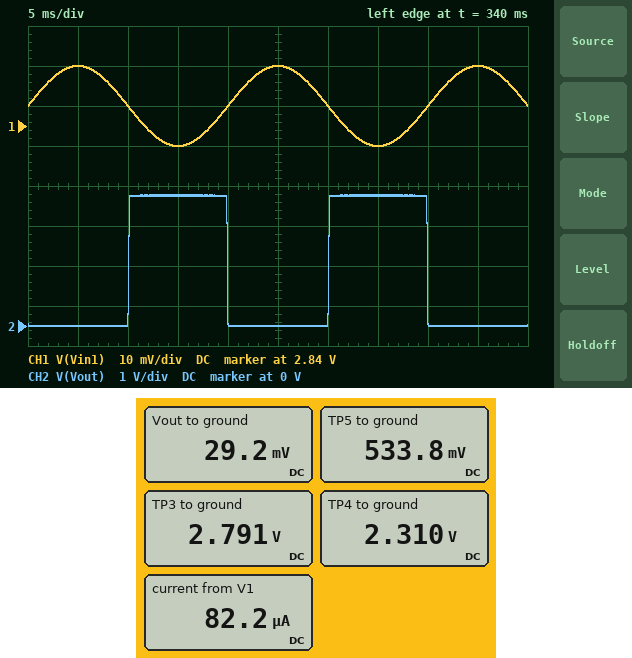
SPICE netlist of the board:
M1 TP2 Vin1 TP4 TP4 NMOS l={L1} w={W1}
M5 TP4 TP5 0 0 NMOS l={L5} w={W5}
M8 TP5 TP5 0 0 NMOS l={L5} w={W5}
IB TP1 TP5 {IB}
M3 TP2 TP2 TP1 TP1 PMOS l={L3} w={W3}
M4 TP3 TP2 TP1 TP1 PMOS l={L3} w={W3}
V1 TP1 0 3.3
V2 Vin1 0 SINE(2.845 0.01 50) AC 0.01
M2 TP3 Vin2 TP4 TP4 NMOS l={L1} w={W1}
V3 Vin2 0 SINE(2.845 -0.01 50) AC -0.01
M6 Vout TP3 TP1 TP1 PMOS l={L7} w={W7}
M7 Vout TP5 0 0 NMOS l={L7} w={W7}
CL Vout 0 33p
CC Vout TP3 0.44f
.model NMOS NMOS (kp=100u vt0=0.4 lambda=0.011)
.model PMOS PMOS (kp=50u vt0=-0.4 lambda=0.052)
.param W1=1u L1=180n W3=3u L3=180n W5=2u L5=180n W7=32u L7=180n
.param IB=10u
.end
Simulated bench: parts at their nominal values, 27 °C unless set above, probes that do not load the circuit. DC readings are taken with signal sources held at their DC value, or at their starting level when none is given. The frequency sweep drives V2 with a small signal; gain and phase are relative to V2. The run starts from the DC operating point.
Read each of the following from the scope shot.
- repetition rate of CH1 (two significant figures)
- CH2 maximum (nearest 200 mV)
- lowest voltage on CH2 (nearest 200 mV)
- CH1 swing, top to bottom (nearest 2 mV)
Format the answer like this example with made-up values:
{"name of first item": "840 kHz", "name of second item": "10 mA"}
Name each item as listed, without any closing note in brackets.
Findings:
{"repetition rate of CH1": "50 Hz", "CH2 maximum": "3.2 V", "lowest voltage on CH2": "0 V", "CH1 swing, top to bottom": "20 mV"}
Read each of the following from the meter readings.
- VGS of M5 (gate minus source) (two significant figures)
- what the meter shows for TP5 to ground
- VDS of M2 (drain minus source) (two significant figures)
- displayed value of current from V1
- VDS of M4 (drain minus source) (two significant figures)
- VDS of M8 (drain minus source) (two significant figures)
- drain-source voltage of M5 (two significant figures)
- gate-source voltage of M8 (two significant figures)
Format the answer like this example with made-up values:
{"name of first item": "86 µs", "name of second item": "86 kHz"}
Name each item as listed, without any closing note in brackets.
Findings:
{"VGS of M5 (gate minus source)": "530 mV", "what the meter shows for TP5 to ground": "533.8 mV", "VDS of M2 (drain minus source)": "480 mV", "displayed value of current from V1": "82.2 µA", "VDS of M4 (drain minus source)": "-510 mV", "VDS of M8 (drain minus source)": "530 mV", "drain-source voltage of M5": "2.3 V", "gate-source voltage of M8": "530 mV"}
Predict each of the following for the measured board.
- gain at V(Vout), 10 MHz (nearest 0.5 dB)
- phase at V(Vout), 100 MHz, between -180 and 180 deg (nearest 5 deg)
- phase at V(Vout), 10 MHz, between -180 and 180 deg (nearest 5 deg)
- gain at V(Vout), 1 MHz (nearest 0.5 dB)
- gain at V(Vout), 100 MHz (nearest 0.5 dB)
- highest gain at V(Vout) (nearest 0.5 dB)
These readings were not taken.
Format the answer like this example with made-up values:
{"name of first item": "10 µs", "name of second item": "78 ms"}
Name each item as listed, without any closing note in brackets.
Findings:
{"gain at V(Vout), 10 MHz": "39.5 dB", "phase at V(Vout), 100 MHz, between -180 and 180 deg": "55 deg", "phase at V(Vout), 10 MHz, between -180 and 180 deg": "125 deg", "gain at V(Vout), 1 MHz": "43.5 dB", "gain at V(Vout), 100 MHz": "19.5 dB", "highest gain at V(Vout)": "43.5 dB"}
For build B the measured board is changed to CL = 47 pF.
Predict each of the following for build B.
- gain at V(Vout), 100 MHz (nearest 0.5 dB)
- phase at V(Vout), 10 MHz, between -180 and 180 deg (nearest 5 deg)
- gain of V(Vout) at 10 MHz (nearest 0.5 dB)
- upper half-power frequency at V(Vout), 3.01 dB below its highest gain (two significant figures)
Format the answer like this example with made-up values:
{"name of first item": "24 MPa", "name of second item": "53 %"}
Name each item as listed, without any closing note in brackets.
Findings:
{"gain at V(Vout), 100 MHz": "16.5 dB", "phase at V(Vout), 10 MHz, between -180 and 180 deg": "115 deg", "gain of V(Vout) at 10 MHz": "37.5 dB", "upper half-power frequency at V(Vout), 3.01 dB below its highest gain": "6.1 MHz"}
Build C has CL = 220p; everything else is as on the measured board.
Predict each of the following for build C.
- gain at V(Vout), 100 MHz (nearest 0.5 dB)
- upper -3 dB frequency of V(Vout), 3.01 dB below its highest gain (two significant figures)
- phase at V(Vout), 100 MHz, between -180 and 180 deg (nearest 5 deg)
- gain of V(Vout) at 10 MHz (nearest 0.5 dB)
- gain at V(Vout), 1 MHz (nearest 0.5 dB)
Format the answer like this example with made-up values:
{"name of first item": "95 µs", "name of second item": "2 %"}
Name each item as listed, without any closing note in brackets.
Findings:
{"gain at V(Vout), 100 MHz": "3.5 dB", "upper -3 dB frequency of V(Vout), 3.01 dB below its highest gain": "1.3 MHz", "phase at V(Vout), 100 MHz, between -180 and 180 deg": "50 deg", "gain of V(Vout) at 10 MHz": "26.0 dB", "gain at V(Vout), 1 MHz": "41.5 dB"}
